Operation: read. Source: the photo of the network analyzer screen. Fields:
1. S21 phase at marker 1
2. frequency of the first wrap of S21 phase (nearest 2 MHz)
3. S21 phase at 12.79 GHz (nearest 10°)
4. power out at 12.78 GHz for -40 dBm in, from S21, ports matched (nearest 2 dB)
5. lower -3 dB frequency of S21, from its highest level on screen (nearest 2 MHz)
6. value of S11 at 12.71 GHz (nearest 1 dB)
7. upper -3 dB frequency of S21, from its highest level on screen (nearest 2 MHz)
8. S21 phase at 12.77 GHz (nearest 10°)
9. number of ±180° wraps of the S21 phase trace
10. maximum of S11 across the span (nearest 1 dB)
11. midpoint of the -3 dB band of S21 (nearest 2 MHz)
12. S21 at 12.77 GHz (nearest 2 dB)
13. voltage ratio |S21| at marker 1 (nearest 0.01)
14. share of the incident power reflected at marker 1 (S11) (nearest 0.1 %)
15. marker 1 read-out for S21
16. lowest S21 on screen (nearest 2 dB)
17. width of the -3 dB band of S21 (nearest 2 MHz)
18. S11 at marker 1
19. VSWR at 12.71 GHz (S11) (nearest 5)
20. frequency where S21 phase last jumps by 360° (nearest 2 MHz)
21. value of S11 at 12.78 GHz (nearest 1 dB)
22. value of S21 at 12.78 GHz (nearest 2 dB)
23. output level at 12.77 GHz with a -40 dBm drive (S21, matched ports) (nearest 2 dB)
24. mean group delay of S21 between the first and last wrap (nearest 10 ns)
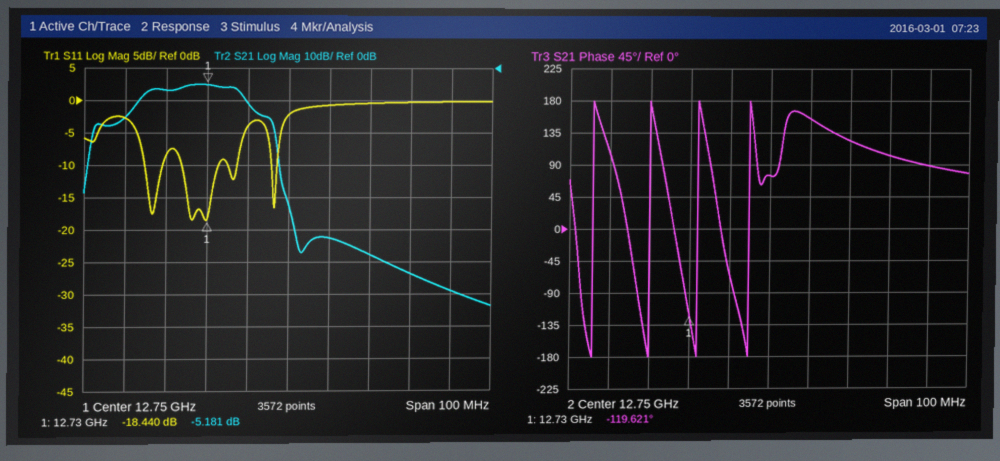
-119.621°
12.706 GHz
90°
-104 dBm
12.714 GHz
-3 dB
12.738 GHz
120°
4
0 dB
12.726 GHz
-58 dB
0.55
1.4 %
-5.181 dB
-74 dB
24 MHz
-18.440 dB
5
12.744 GHz
0 dB
-64 dB
-98 dBm
80 ns
